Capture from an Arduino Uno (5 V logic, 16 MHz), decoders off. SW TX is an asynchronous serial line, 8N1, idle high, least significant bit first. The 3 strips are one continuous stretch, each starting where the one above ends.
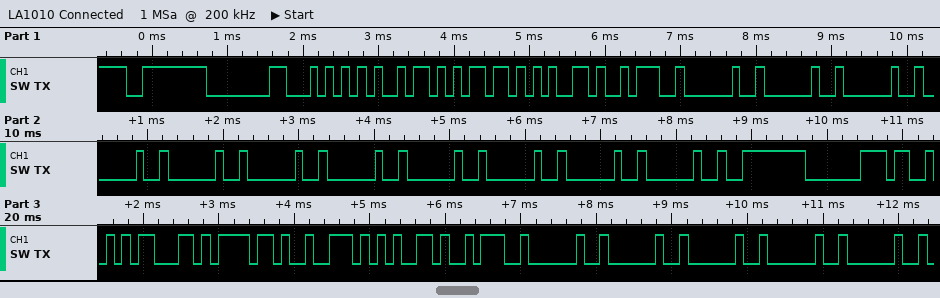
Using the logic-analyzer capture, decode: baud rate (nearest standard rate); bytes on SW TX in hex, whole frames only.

9600 baud
FE 80 54 69 6D 65 3A 20 20 20 20 20 20 20 20 20 20 20 FE C0 53 63 6F 72 65 3A 20 20 20 20 20
